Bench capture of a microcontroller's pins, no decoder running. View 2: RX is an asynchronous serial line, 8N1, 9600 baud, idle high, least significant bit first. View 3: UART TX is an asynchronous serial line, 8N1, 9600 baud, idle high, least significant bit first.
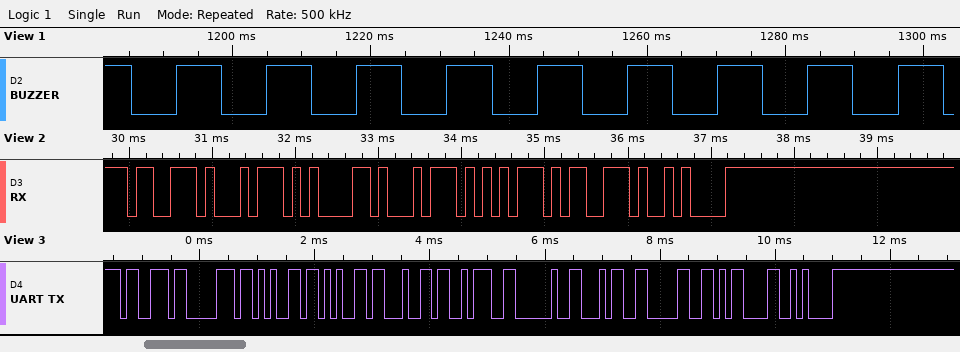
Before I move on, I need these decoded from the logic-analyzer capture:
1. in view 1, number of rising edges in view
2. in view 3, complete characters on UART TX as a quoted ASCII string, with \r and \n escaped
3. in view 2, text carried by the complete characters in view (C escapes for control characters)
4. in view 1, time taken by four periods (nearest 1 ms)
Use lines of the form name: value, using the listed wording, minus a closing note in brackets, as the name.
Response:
in view 1, number of rising edges in view: 9
in view 3, complete characters on UART TX as a quoted ASCII string, with \r and \n escaped: "speed: 40\r\n"
in view 2, text carried by the complete characters in view: "status\n"
in view 1, time taken by four periods: 52 ms
